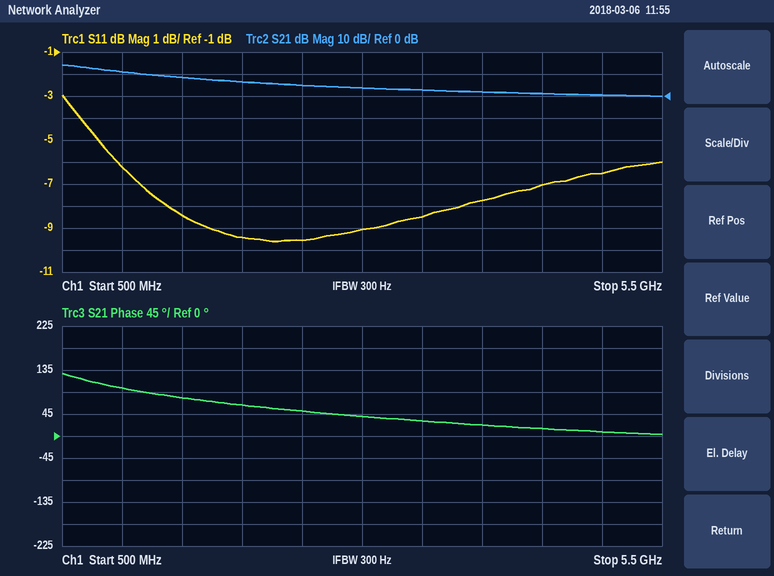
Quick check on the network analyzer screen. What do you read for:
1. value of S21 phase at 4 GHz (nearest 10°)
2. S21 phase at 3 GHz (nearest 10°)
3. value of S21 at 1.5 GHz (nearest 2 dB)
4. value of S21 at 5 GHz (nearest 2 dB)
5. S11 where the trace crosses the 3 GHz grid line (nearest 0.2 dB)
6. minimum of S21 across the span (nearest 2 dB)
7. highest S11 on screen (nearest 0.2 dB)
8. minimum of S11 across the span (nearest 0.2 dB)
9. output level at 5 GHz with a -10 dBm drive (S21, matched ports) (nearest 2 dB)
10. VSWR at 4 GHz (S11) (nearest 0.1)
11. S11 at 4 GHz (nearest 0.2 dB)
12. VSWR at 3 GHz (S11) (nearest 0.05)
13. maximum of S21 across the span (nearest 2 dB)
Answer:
20°
40°
8 dB
0 dB
-9.0 dB
0 dB
-3.0 dB
-9.6 dB
-10 dBm
2.4
-7.8 dB
2.10
14 dB
